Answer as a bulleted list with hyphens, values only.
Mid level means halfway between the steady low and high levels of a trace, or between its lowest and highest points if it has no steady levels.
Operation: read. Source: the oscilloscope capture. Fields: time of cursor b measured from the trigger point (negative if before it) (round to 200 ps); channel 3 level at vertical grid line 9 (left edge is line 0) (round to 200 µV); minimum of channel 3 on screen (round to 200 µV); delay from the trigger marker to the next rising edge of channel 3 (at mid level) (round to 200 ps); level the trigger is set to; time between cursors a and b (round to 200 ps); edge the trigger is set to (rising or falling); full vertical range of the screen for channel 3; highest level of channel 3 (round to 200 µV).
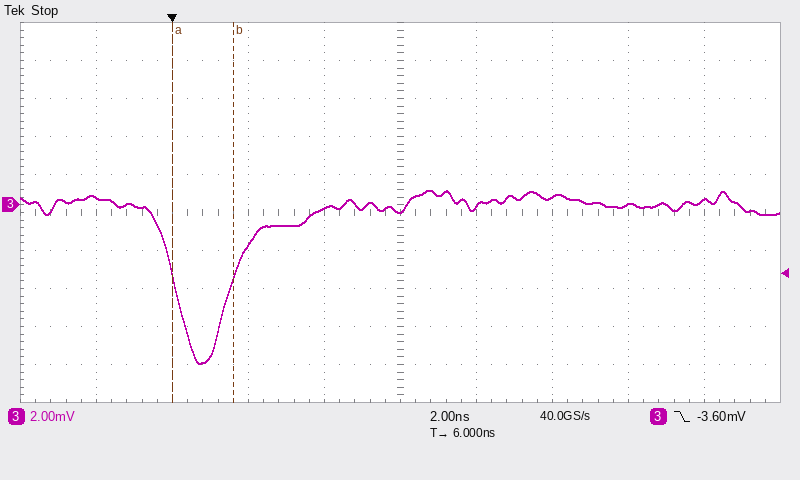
- +1.6 ns
- 200 µV
- -8.4 mV
- 1.6 ns
- -3.60 mV
- 1.6 ns
- falling
- 20 mV
- 800 µV
